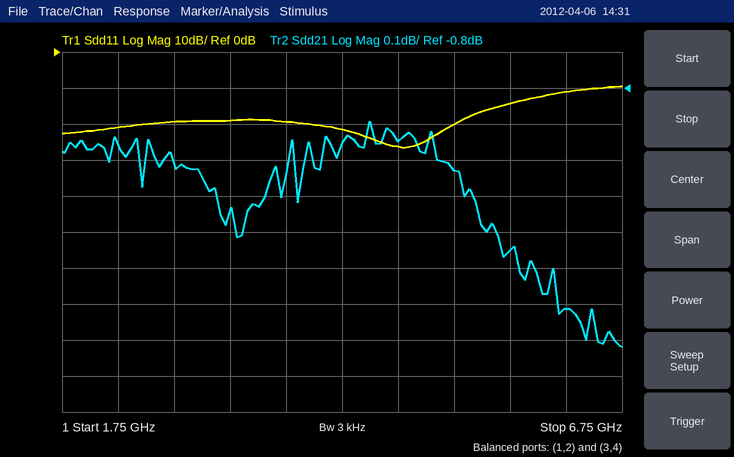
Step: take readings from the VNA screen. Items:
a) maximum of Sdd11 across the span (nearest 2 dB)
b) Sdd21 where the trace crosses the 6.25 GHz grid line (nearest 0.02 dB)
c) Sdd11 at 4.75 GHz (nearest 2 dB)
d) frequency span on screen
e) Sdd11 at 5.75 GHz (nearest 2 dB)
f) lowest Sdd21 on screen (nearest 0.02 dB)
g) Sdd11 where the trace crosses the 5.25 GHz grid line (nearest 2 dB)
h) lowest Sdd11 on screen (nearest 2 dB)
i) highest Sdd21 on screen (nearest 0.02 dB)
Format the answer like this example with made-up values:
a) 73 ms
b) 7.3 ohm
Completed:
a) -10 dB
b) -1.42 dB
c) -26 dB
d) 5 GHz
e) -14 dB
f) -1.52 dB
g) -20 dB
h) -26 dB
i) -0.90 dB
